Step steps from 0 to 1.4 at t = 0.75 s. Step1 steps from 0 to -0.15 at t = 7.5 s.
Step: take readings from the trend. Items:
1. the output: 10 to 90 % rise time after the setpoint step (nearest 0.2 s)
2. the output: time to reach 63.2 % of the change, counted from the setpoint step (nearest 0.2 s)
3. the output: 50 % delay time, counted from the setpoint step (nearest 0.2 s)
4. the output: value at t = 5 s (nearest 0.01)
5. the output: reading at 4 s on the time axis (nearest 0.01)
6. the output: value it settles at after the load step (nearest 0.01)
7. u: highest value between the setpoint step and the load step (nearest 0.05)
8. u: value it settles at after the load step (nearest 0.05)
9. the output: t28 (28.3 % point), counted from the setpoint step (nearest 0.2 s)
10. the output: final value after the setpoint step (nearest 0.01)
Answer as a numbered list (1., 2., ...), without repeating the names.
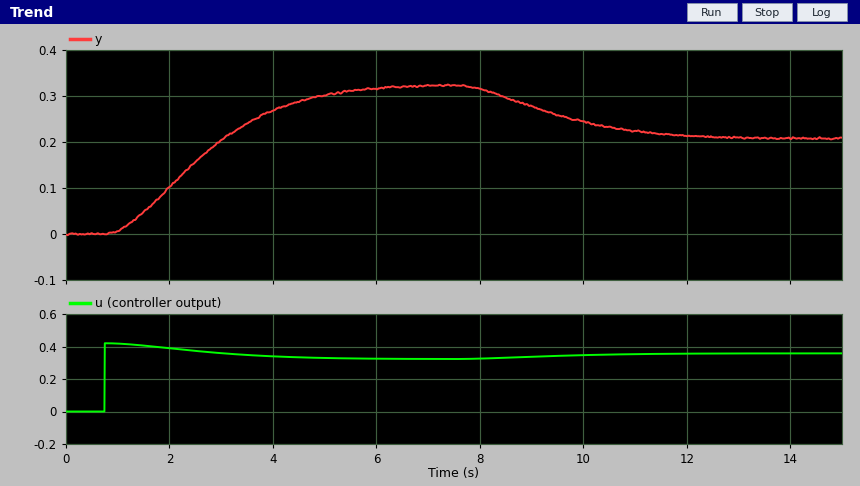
1. 3.2 s
2. 2.2 s
3. 1.8 s
4. 0.30
5. 0.27
6. 0.21
7. 0.40
8. 0.35
9. 1.2 s
10. 0.32
